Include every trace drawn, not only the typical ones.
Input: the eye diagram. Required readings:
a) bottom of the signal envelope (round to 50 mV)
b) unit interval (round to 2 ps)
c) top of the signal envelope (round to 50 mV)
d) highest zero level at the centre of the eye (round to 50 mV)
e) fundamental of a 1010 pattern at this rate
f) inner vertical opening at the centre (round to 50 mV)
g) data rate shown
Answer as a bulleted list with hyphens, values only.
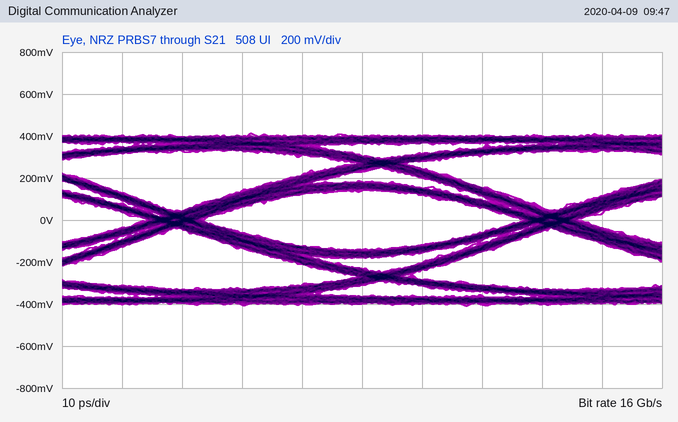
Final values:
- -400 mV
- 62 ps
- 400 mV
- -150 mV
- 8 GHz
- 300 mV
- 16 Gb/s
